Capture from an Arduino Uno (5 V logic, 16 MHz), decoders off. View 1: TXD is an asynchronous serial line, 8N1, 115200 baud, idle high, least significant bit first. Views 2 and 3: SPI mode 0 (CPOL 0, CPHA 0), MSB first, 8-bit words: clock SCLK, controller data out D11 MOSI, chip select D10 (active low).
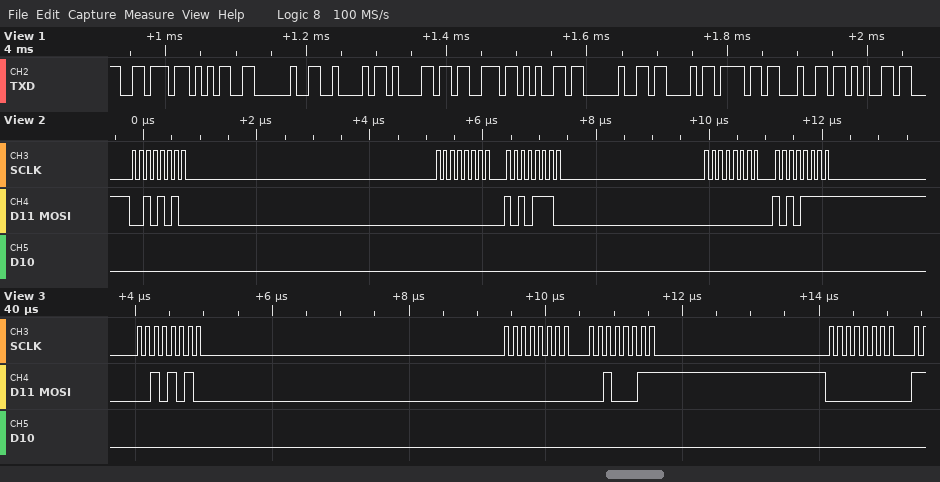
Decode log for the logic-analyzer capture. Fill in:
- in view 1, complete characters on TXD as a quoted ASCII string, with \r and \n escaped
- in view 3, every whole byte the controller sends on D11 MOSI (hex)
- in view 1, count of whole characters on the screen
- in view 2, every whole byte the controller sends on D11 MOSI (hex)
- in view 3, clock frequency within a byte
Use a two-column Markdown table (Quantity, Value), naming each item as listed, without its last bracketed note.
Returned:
| Quantity | Value |
|---|---|
| in view 1, complete characters on TXD as a quoted ASCII string, with \r and \n escaped | "v5 Base Code" |
| in view 3, every whole byte the controller sends on D11 MOSI | 2A 00 23 00 |
| in view 1, count of whole characters on the screen | 12 |
| in view 2, every whole byte the controller sends on D11 MOSI | 2A 00 AE 00 AF |
| in view 3, clock frequency within a byte | 8 MHz |
